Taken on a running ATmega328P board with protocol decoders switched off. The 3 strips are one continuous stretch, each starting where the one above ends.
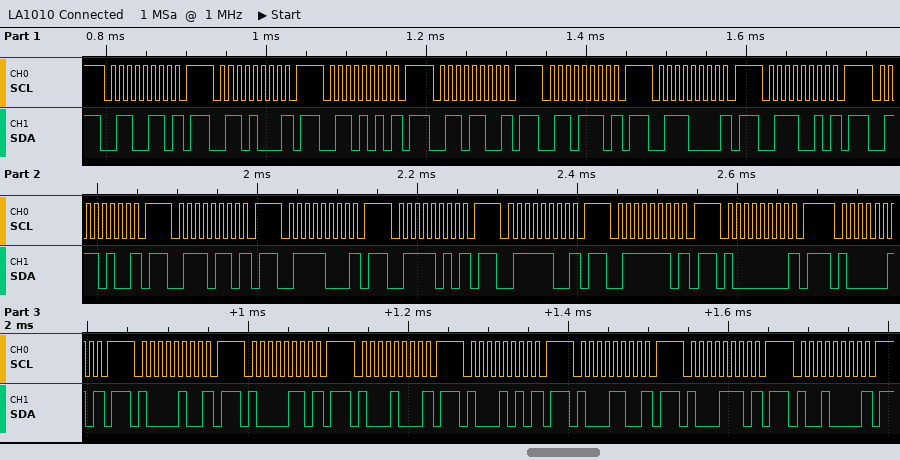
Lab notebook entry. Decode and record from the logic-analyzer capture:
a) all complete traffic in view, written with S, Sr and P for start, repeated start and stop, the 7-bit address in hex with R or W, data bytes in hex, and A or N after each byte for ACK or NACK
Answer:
S 33W N P S 34W N P S 35W N P S 36W N P S 37W N P S 38W N P S 39W N P S 3AW N P S 3BW N P S 3CW N P S 3DW N P S 3EW N P S 3FW N P S 40W N P S 41W N P S 42W N P S 43W N P S 44W N P S 45W N P S 46W N P S 47W N P S 48W N P
